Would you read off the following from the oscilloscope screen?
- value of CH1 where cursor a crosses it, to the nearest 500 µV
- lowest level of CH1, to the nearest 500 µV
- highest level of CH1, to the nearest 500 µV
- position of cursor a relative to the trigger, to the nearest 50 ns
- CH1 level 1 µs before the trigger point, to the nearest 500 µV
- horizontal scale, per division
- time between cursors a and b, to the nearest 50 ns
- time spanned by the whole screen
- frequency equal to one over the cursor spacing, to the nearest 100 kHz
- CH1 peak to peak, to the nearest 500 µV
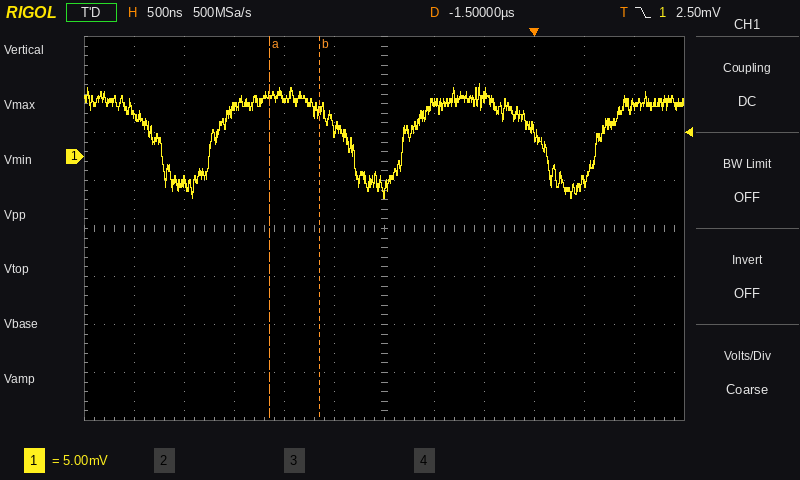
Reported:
6.5 mV
-4.5 mV
7.5 mV
-2.65 µs
5.5 mV
500 ns
500 ns
6 µs
2.0 MHz
12.0 mV
